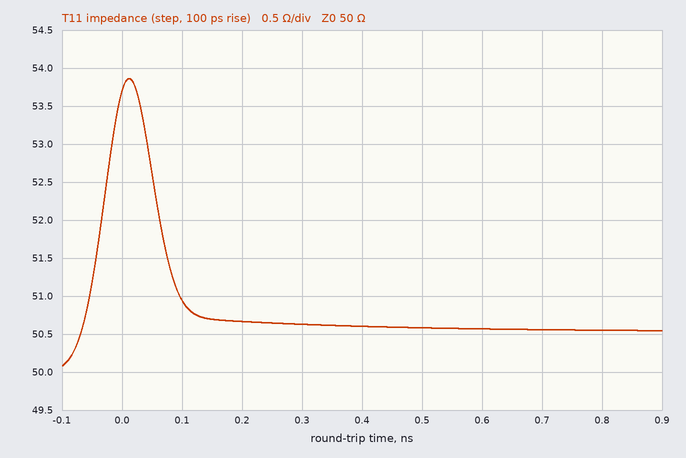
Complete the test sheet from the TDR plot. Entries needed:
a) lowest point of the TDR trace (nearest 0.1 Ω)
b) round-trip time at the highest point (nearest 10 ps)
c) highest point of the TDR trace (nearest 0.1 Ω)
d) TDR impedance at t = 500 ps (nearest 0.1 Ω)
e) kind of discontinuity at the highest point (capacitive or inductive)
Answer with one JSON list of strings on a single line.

["50.1 Ω", "10 ps", "53.9 Ω", "50.6 Ω", "inductive"]
